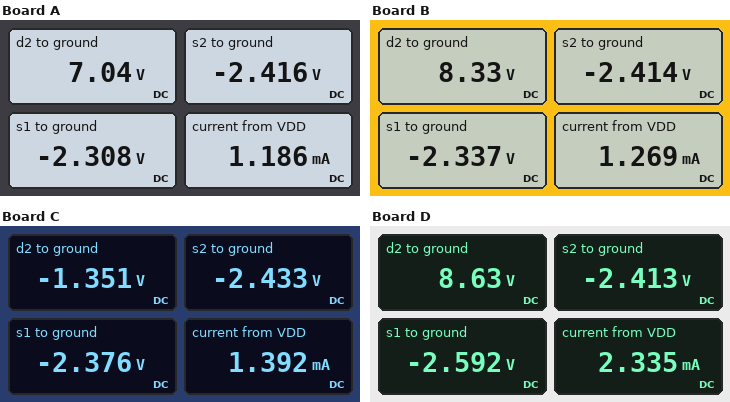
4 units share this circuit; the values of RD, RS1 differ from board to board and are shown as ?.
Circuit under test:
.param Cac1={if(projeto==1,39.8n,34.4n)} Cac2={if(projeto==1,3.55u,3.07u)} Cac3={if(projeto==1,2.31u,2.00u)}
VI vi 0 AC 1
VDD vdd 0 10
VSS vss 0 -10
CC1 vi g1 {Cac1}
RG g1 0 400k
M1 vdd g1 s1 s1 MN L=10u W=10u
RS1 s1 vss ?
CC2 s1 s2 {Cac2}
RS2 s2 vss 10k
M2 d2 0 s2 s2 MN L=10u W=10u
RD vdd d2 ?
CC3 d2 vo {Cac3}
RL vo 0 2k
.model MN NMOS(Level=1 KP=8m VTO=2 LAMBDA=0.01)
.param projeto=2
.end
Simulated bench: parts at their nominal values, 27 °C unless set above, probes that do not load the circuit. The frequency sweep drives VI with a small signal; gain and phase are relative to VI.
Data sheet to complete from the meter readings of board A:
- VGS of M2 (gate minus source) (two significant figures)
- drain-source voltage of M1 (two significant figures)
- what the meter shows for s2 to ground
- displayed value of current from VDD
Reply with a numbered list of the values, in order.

1. 2.4 V
2. 12 V
3. -2.416 V
4. 1.186 mA
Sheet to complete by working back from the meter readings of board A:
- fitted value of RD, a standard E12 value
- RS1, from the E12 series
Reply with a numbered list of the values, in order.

1. 3.9 kΩ
2. 18 kΩ
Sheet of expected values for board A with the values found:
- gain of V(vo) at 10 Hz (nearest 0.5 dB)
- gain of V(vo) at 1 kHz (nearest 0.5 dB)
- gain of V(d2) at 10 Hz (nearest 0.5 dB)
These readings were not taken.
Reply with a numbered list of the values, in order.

1. -20.5 dB
2. 6.0 dB
3. -8.5 dB
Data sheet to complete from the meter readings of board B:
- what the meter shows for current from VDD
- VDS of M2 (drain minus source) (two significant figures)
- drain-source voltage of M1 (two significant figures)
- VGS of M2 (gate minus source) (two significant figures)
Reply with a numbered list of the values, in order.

1. 1.269 mA
2. 11 V
3. 12 V
4. 2.4 V
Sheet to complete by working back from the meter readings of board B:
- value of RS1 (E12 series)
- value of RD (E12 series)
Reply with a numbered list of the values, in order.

1. 15 kΩ
2. 2.2 kΩ
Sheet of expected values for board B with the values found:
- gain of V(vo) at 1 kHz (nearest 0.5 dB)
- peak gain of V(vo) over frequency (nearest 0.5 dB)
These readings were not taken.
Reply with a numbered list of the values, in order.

1. 4.5 dB
2. 4.5 dB
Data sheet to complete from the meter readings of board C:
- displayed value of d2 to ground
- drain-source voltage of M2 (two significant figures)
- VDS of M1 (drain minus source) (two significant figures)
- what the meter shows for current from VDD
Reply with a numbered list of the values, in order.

1. -1.351 V
2. 1.1 V
3. 12 V
4. 1.392 mA
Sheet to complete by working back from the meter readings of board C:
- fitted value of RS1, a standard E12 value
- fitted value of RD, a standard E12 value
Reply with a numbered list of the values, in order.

1. 12 kΩ
2. 15 kΩ
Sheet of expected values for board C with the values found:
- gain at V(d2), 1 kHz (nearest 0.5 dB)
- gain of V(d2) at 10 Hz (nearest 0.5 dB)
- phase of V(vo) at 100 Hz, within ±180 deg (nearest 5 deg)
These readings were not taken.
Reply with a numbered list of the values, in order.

1. 9.5 dB
2. -2.0 dB
3. 50 deg
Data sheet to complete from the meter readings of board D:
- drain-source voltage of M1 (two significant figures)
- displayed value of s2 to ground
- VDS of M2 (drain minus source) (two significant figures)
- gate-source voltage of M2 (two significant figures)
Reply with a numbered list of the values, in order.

1. 13 V
2. -2.413 V
3. 11 V
4. 2.4 V
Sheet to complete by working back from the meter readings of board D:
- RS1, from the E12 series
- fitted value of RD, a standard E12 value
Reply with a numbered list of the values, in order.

1. 4.7 kΩ
2. 1.8 kΩ
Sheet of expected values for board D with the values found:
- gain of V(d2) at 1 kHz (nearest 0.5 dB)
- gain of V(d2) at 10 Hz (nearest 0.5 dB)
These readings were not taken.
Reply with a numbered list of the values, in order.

1. 6.0 dB
2. -14.0 dB
